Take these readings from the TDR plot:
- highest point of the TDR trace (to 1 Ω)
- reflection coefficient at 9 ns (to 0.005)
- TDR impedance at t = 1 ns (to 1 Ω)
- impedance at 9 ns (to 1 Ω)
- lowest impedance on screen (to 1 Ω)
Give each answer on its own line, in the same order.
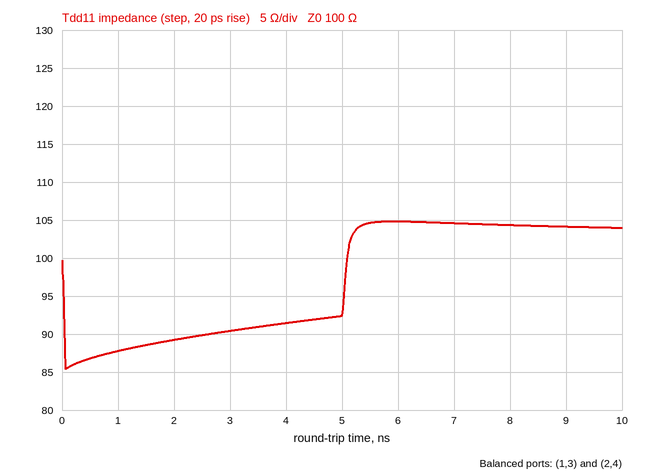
105 Ω
+0.020
88 Ω
104 Ω
85 Ω
